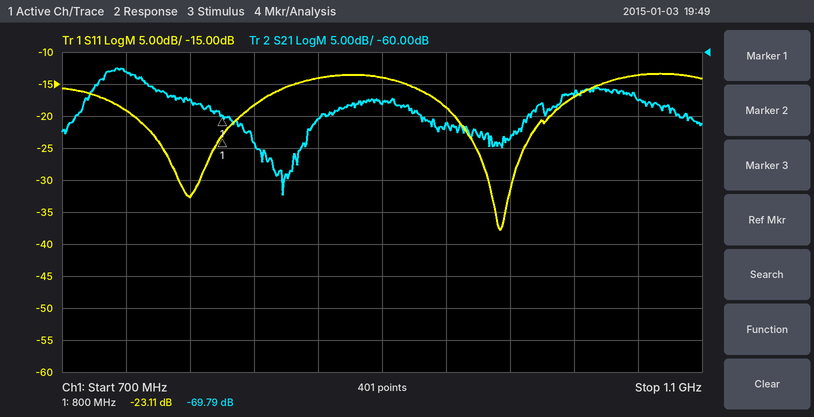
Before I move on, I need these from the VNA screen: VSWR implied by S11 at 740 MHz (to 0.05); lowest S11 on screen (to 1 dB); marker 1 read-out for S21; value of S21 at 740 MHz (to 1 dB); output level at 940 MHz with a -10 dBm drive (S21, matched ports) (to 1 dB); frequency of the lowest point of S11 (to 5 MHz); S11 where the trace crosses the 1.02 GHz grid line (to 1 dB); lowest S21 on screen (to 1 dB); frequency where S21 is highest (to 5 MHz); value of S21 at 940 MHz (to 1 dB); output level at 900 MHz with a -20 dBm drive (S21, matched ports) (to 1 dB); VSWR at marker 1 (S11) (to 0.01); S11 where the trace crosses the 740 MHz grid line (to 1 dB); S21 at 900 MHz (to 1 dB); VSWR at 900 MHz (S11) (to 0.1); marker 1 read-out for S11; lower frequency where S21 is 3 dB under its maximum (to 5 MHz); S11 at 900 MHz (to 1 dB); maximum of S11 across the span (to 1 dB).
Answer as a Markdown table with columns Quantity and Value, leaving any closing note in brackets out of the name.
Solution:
| Quantity | Value |
|---|---|
| VSWR implied by S11 at 740 MHz | 1.25 |
| lowest S11 on screen | -38 dB |
| marker 1 read-out for S21 | -69.79 dB |
| value of S21 at 740 MHz | -63 dB |
| output level at 940 MHz with a -10 dBm drive (S21, matched ports) | -81 dBm |
| frequency of the lowest point of S11 | 975 MHz |
| S11 where the trace crosses the 1.02 GHz grid line | -17 dB |
| lowest S21 on screen | -82 dB |
| frequency where S21 is highest | 735 MHz |
| value of S21 at 940 MHz | -71 dB |
| output level at 900 MHz with a -20 dBm drive (S21, matched ports) | -88 dBm |
| VSWR at marker 1 (S11) | 1.15 |
| S11 where the trace crosses the 740 MHz grid line | -19 dB |
| S21 at 900 MHz | -68 dB |
| VSWR at 900 MHz (S11) | 1.5 |
| marker 1 read-out for S11 | -23.11 dB |
| lower frequency where S21 is 3 dB under its maximum | 720 MHz |
| S11 at 900 MHz | -14 dB |
| maximum of S11 across the span | -13 dB |
